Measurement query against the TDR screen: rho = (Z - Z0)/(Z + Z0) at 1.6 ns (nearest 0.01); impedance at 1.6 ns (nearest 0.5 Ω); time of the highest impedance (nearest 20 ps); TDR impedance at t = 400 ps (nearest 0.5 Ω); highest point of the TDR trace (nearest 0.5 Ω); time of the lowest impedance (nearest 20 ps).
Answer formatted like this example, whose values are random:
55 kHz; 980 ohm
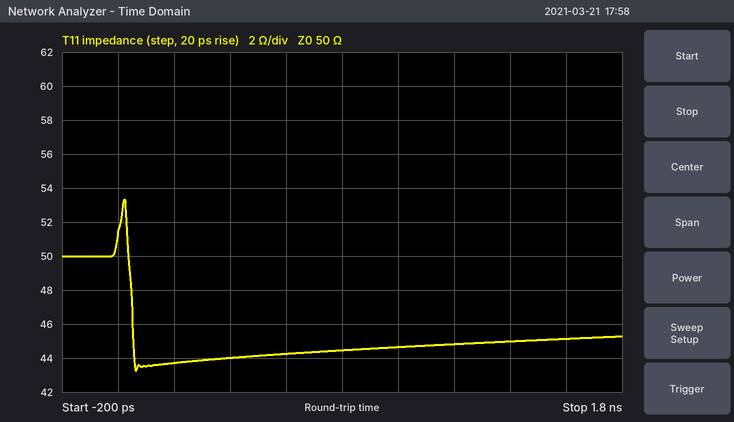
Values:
-0.05; 45.0 Ω; 20 ps; 44.0 Ω; 53.5 Ω; 60 ps
